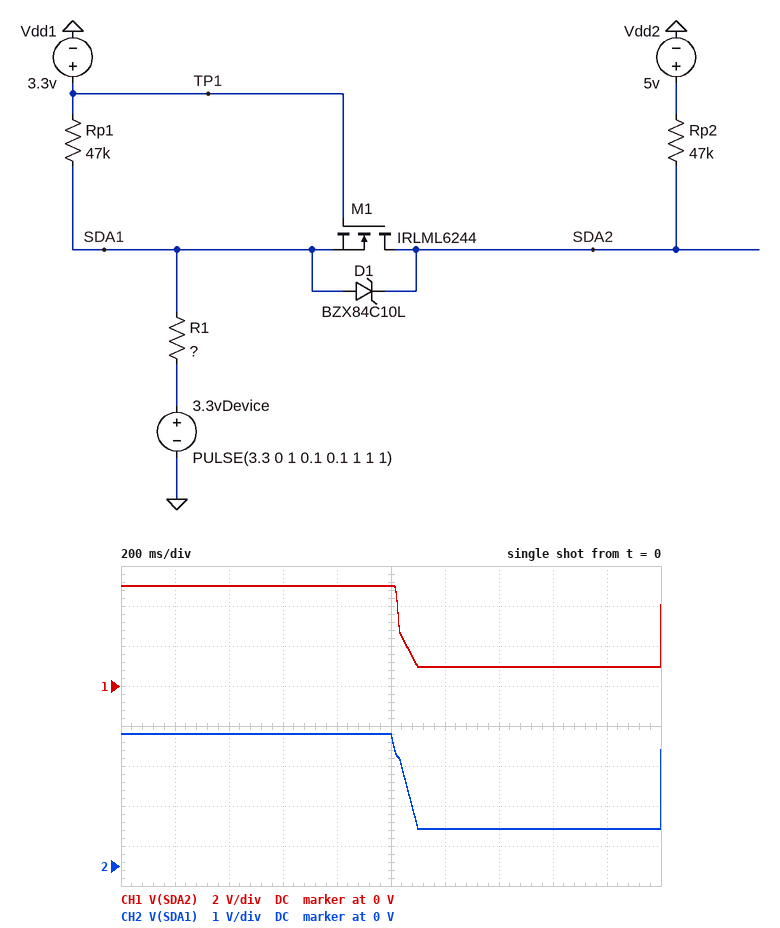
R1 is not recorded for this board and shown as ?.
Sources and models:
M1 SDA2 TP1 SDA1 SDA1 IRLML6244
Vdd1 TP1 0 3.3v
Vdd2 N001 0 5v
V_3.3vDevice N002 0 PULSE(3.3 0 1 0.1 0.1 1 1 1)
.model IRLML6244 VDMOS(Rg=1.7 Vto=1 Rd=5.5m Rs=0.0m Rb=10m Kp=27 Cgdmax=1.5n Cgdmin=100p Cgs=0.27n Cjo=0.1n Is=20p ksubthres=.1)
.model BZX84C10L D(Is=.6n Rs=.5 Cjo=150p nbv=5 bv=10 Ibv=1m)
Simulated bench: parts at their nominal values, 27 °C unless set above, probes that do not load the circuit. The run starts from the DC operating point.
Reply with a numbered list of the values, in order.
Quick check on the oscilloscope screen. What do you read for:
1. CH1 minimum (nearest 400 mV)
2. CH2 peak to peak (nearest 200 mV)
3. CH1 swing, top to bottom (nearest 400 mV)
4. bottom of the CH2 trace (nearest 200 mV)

1. 800 mV
2. 2.4 V
3. 4.0 V
4. 1.0 V
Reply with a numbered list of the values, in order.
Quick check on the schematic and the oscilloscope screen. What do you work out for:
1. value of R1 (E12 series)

1. 6.8 kΩ
